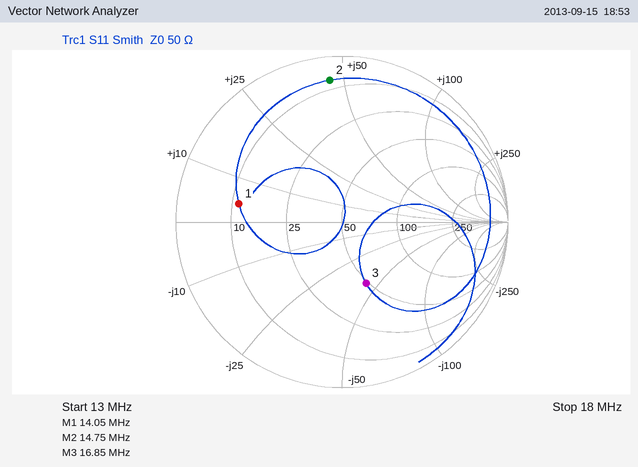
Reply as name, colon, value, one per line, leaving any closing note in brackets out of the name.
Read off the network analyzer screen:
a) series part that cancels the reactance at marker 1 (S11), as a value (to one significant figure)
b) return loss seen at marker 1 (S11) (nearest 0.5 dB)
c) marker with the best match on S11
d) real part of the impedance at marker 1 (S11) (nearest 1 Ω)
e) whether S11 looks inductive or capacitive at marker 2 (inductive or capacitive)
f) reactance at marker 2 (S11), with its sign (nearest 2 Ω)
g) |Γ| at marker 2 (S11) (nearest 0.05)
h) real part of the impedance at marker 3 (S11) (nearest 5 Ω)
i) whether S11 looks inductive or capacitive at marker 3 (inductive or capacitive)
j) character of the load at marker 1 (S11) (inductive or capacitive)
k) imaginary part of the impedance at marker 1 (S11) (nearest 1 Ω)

series part that cancels the reactance at marker 1 (S11), as a value: 3 nF
return loss seen at marker 1 (S11): 4.0 dB
marker with the best match on S11: marker 3
real part of the impedance at marker 1 (S11): 11 Ω
whether S11 looks inductive or capacitive at marker 2: inductive
reactance at marker 2 (S11), with its sign: +46 Ω
|Γ| at marker 2 (S11): 0.85
real part of the impedance at marker 3 (S11): 50 Ω
whether S11 looks inductive or capacitive at marker 3: capacitive
character of the load at marker 1 (S11): inductive
imaginary part of the impedance at marker 1 (S11): +4 Ω
